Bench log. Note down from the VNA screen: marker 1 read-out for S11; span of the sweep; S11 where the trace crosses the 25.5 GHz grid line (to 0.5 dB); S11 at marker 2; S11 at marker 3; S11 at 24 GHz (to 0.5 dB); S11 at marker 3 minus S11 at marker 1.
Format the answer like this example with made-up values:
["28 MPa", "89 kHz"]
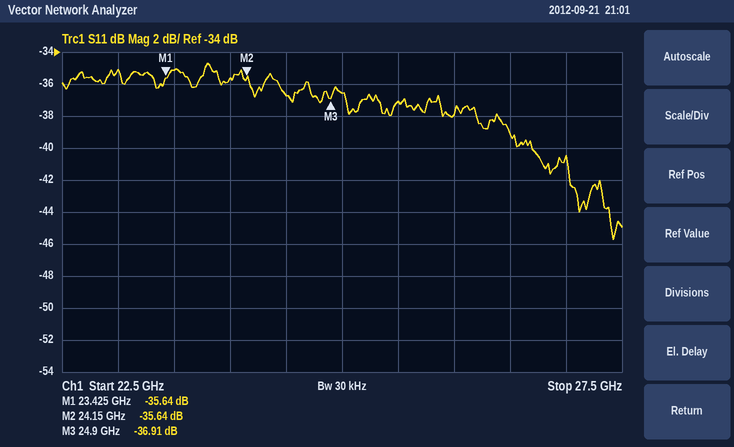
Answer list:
["-35.64 dB", "5 GHz", "-37.0 dB", "-35.64 dB", "-36.91 dB", "-35.5 dB", "-1.27 dB"]
